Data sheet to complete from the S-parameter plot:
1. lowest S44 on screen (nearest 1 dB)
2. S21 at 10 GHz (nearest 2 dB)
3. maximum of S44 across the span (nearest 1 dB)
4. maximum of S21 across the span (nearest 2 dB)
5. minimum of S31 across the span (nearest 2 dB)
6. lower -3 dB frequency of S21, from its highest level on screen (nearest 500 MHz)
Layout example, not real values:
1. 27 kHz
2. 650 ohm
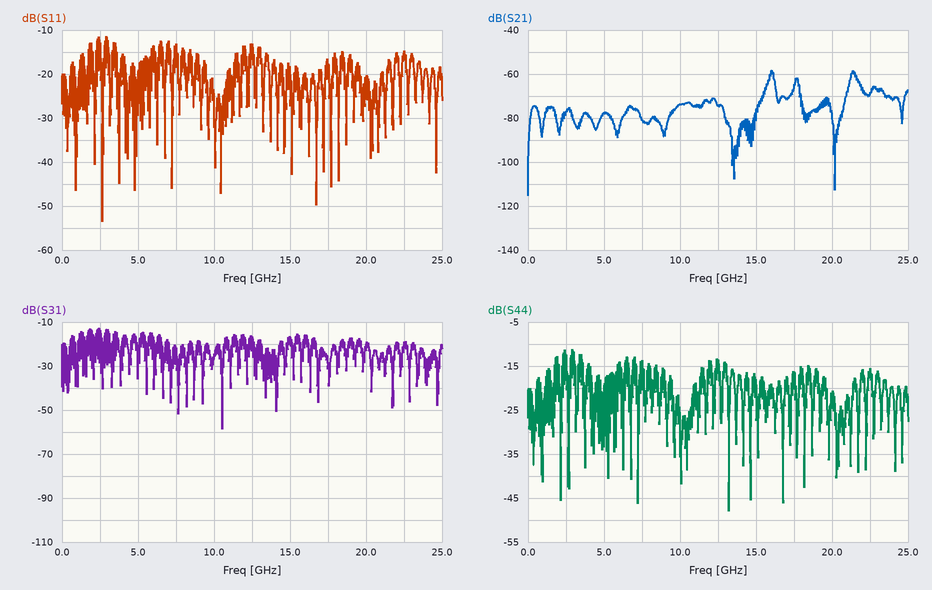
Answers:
1. -48 dB
2. -74 dB
3. -11 dB
4. -58 dB
5. -58 dB
6. 16.0 GHz
